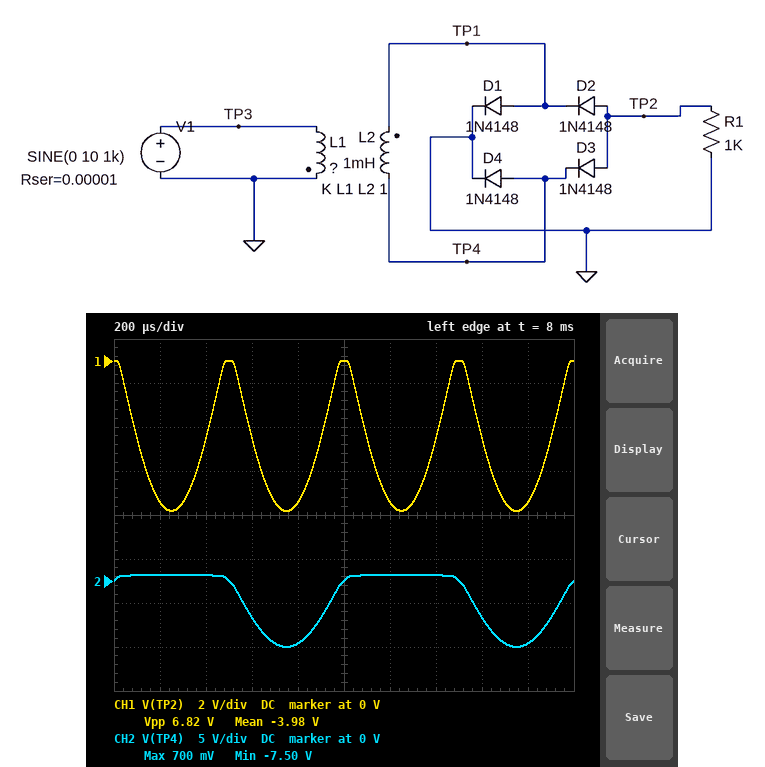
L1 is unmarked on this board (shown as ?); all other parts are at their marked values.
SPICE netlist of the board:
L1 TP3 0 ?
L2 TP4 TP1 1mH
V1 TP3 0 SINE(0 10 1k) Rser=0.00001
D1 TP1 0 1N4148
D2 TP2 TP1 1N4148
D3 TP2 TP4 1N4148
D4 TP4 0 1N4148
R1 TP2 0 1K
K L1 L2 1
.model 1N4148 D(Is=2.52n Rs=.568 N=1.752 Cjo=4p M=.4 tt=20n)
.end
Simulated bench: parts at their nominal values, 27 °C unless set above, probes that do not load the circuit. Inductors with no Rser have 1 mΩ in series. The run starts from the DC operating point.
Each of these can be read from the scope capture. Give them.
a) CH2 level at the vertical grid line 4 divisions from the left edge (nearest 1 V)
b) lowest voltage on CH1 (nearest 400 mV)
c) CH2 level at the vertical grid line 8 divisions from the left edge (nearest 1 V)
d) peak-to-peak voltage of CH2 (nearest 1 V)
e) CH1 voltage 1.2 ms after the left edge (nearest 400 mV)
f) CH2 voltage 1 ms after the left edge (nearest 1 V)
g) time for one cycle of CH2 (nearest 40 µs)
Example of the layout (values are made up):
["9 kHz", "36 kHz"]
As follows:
["-7 V", "-6.8 V", "-4 V", "8 V", "-6.4 V", "0 V", "1.00 ms"]
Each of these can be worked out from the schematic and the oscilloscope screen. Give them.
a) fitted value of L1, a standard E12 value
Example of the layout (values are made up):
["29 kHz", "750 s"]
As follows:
["1.5 mH"]
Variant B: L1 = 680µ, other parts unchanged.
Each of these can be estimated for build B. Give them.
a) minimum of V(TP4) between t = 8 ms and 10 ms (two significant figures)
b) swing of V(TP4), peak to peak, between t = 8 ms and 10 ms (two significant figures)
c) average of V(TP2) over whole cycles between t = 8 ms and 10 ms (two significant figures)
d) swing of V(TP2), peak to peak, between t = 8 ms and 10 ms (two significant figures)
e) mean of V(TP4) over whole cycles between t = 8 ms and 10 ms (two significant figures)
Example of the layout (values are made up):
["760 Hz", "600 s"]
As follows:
["-11 V", "12 V", "-6.4 V", "11 V", "-3.2 V"]
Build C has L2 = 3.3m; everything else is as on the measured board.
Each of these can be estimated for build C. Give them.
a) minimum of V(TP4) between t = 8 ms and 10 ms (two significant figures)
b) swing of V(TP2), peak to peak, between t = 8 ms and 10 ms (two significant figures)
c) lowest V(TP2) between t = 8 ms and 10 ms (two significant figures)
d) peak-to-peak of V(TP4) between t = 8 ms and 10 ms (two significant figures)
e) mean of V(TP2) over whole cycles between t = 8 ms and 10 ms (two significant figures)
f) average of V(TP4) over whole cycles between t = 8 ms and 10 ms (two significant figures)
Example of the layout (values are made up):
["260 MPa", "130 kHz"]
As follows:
["-14 V", "13 V", "-13 V", "15 V", "-8.1 V", "-4.1 V"]
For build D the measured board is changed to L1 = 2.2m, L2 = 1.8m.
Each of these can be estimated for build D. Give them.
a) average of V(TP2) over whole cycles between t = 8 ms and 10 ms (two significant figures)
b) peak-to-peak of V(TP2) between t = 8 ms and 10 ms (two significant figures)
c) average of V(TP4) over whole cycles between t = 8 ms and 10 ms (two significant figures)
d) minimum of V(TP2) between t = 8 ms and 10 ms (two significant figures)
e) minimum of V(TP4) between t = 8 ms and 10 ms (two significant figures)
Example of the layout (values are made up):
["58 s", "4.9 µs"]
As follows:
["-4.5 V", "7.7 V", "-2.3 V", "-7.7 V", "-8.4 V"]
